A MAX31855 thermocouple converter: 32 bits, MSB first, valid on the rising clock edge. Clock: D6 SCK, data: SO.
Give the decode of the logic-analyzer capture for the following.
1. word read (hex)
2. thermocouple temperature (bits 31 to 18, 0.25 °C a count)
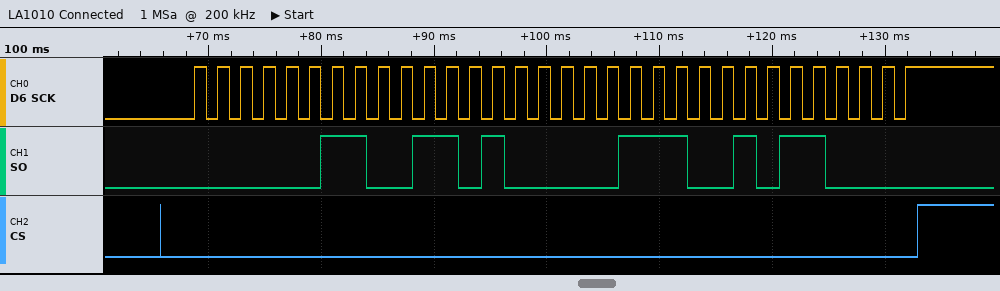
0x03341CB0
51.25 °C
